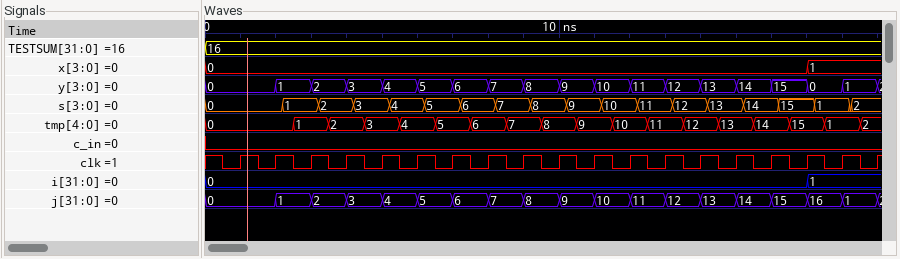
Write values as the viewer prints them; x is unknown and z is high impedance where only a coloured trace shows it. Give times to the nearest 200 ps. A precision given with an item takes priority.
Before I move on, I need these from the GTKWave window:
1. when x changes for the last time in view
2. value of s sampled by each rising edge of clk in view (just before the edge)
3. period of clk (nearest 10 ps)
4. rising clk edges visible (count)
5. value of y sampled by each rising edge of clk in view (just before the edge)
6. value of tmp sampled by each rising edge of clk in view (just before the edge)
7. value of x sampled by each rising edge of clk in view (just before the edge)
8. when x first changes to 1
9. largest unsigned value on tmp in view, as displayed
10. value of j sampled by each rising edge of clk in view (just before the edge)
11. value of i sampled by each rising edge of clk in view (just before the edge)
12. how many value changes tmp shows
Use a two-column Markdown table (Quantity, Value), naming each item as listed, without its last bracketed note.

| Quantity | Value |
|---|---|
| when x changes for the last time in view | 17000 ps |
| value of s sampled by each rising edge of clk in view | 0, 0, 1, 2, 3, 4, 5, 6, 7, 8, 9, 10, 11, 12, 13, 14, 15, 1, 2 |
| period of clk | 1000 ps |
| rising clk edges visible | 19 |
| value of y sampled by each rising edge of clk in view | 0, 0, 1, 2, 3, 4, 5, 6, 7, 8, 9, 10, 11, 12, 13, 14, 15, 0, 1 |
| value of tmp sampled by each rising edge of clk in view | 0, 0, 1, 2, 3, 4, 5, 6, 7, 8, 9, 10, 11, 12, 13, 14, 15, 1, 2 |
| value of x sampled by each rising edge of clk in view | 0, 0, 0, 0, 0, 0, 0, 0, 0, 0, 0, 0, 0, 0, 0, 0, 0, 1, 1 |
| when x first changes to 1 | 17000 ps |
| largest unsigned value on tmp in view, as displayed | 15 |
| value of j sampled by each rising edge of clk in view | 0, 0, 1, 2, 3, 4, 5, 6, 7, 8, 9, 10, 11, 12, 13, 14, 15, 16, 1 |
| value of i sampled by each rising edge of clk in view | 0, 0, 0, 0, 0, 0, 0, 0, 0, 0, 0, 0, 0, 0, 0, 0, 0, 1, 1 |
| how many value changes tmp shows | 17 |
